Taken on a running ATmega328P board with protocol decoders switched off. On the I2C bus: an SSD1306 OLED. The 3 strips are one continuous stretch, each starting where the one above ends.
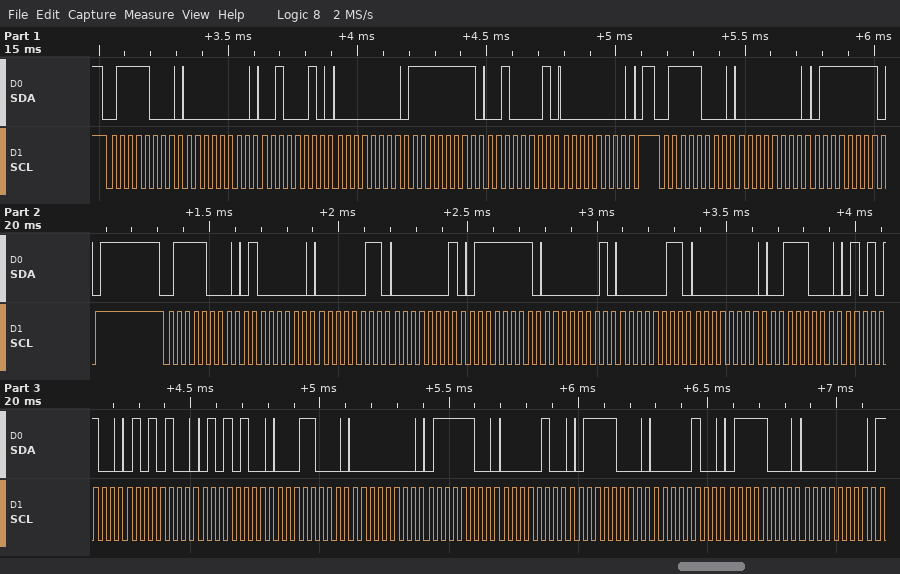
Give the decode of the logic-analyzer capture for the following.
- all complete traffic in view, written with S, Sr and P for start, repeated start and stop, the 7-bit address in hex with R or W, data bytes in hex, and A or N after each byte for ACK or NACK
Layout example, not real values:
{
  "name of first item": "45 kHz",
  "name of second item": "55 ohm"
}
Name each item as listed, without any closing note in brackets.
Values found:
{
  "all complete traffic in view, written with S, Sr and P for start, repeated start and stop, the 7-bit address in hex with R or W, data bytes in hex, and A or N after each byte for ACK or NACK": "S 3CW A 00 A 22 A 00 A FF A 21 A 00 A P S 3CW A 00 A 7F A P S 3CW A 40 A 03 A 01 A 7F A 01 A 03 A 00 A 38 A 54 A 54 A 54 A 18 A 00 A 7C A 04 A 78 A 04 A 78 A 00 A"
}
